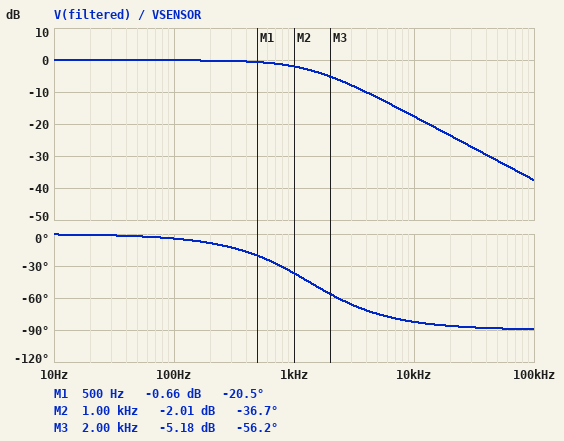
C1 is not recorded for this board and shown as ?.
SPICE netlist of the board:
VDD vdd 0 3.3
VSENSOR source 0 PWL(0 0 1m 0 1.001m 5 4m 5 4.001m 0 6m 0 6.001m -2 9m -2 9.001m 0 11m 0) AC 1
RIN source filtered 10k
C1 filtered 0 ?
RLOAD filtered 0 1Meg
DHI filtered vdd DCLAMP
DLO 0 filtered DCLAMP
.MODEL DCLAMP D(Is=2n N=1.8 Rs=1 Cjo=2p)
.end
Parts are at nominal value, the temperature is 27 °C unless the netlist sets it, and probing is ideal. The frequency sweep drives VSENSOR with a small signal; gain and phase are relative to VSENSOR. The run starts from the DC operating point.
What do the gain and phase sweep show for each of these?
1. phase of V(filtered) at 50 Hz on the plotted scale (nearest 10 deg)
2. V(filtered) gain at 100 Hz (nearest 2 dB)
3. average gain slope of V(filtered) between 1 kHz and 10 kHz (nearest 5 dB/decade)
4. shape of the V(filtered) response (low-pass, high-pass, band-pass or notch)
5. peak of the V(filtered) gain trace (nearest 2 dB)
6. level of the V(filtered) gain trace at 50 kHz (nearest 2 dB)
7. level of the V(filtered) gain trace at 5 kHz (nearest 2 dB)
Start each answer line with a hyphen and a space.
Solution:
- 0 deg
- 0 dB
- -15 dB/decade
- low-pass
- 0 dB
- -32 dB
- -12 dB
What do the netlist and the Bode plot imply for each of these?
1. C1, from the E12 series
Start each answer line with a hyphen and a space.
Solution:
- 12 nF
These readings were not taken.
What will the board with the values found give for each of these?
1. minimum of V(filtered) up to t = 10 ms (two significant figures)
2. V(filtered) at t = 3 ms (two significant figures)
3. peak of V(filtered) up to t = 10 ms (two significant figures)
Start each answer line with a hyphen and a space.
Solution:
- -520 mV
- 3.8 V
- 3.8 V
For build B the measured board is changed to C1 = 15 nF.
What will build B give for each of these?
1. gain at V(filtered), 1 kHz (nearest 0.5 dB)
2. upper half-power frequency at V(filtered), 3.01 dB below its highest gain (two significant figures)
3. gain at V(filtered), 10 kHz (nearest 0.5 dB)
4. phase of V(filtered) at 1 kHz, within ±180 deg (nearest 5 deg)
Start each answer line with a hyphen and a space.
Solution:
- -3.0 dB
- 1.1 kHz
- -19.5 dB
- -45 deg
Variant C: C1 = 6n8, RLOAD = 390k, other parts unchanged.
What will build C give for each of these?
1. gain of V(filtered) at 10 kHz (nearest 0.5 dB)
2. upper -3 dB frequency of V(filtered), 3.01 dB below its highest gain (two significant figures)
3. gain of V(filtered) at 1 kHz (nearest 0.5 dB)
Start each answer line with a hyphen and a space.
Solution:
- -13.0 dB
- 2.4 kHz
- -1.0 dB
